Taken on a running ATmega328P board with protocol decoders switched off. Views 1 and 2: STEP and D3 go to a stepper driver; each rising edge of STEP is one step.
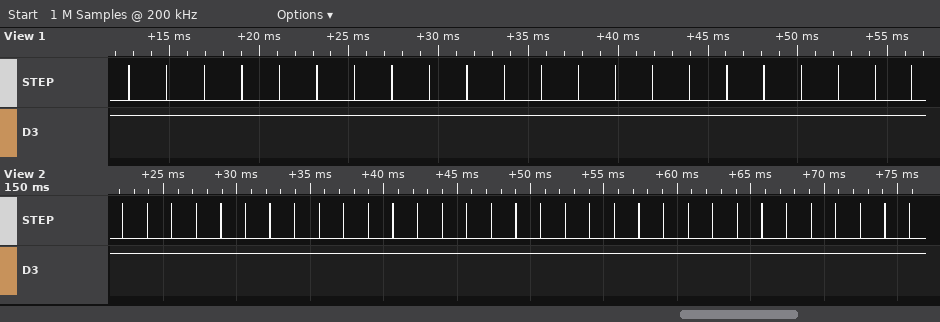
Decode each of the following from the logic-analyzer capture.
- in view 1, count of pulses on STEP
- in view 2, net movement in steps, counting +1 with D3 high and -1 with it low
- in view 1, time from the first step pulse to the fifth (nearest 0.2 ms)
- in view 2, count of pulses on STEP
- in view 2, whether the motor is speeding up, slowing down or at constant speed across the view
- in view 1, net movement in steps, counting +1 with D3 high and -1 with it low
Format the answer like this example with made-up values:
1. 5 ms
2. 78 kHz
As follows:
1. 22
2. +33
3. 8.4 ms
4. 33
5. constant speed
6. +22
